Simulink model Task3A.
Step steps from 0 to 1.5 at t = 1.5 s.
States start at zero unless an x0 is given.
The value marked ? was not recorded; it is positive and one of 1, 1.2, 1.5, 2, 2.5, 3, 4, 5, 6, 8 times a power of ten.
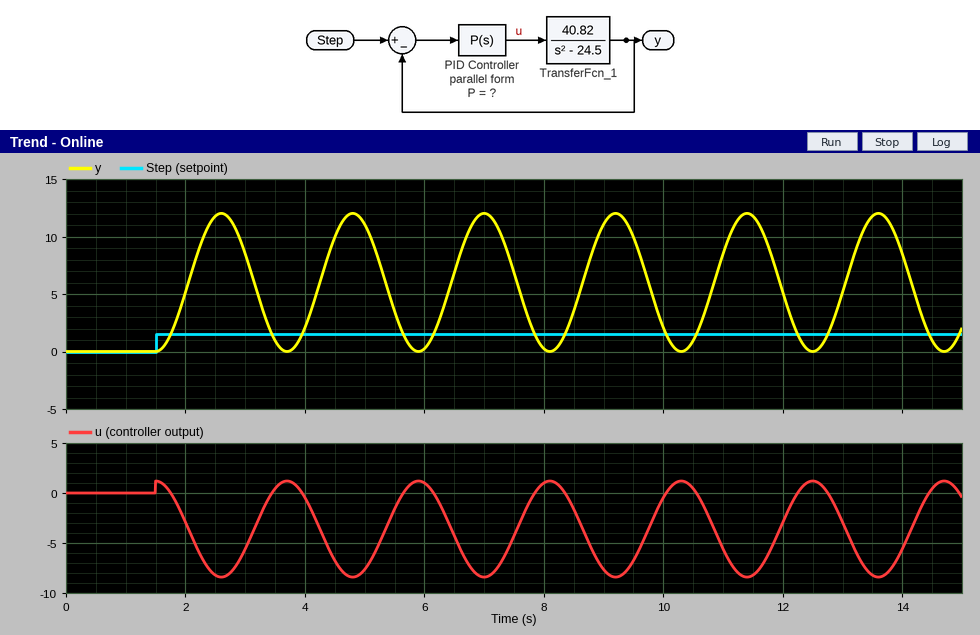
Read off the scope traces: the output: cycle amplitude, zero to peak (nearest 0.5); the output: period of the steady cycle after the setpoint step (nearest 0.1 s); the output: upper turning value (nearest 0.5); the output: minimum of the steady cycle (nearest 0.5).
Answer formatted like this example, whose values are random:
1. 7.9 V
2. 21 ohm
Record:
1. 6.0
2. 2.2 s
3. 12.0
4. 0.0
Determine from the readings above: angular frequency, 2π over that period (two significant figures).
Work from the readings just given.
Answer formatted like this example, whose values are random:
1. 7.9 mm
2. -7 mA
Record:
1. 2.9 rad/s
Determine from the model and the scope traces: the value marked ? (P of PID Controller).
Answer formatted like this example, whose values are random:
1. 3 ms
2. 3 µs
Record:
1. 0.8
